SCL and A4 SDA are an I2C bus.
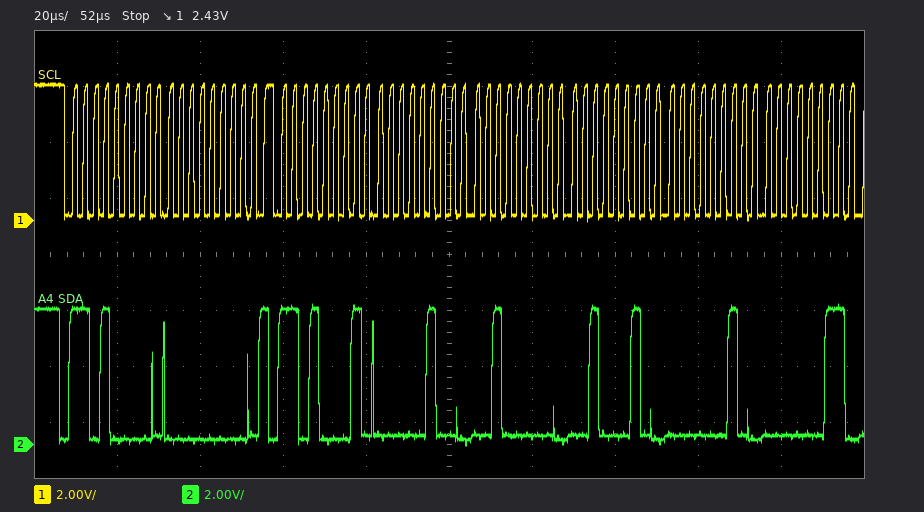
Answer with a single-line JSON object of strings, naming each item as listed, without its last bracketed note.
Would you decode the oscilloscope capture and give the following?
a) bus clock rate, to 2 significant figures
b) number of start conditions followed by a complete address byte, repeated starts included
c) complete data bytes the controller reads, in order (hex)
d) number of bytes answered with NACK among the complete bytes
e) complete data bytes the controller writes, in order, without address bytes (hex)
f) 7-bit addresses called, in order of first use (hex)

{"bus clock rate, to 2 significant figures": "400 kHz", "number of start conditions followed by a complete address byte, repeated starts included": "2", "complete data bytes the controller reads, in order": "04 20 22 02 03", "number of bytes answered with NACK among the complete bytes": "0", "complete data bytes the controller writes, in order, without address bytes": "00", "7-bit addresses called, in order of first use": "0x68"}
